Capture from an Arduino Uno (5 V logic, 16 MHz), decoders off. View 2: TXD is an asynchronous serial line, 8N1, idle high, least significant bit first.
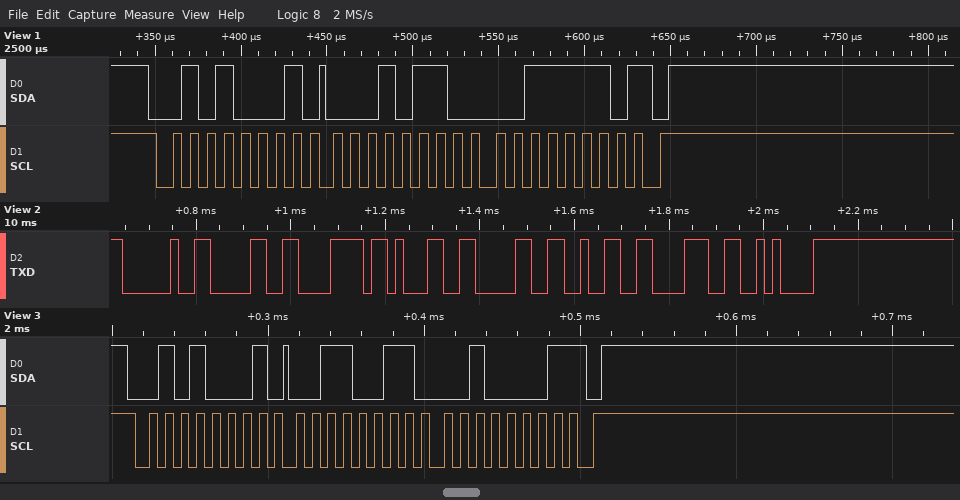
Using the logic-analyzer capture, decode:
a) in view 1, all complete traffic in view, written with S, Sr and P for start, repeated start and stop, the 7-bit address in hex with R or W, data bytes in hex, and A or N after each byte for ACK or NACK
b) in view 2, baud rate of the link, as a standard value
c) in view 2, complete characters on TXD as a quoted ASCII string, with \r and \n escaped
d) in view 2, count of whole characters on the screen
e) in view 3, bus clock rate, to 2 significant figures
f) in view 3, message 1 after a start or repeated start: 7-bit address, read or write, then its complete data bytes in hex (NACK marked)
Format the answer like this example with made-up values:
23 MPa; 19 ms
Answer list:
S 28R A 16 A 3E N P; 57600 baud; " 0x1028\n"; 8; 100 kHz; 0x28 read: 33 21 NACK
